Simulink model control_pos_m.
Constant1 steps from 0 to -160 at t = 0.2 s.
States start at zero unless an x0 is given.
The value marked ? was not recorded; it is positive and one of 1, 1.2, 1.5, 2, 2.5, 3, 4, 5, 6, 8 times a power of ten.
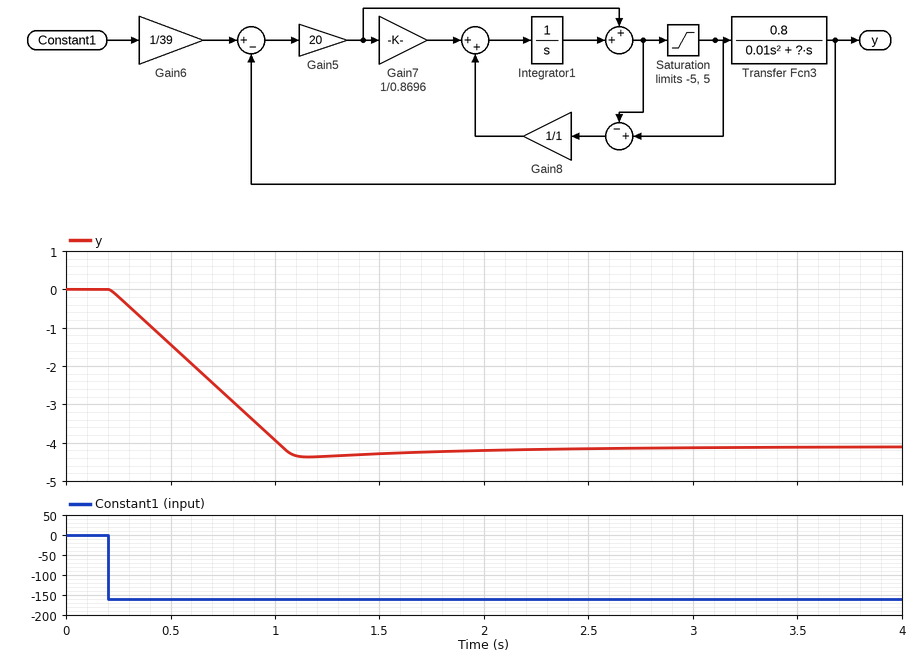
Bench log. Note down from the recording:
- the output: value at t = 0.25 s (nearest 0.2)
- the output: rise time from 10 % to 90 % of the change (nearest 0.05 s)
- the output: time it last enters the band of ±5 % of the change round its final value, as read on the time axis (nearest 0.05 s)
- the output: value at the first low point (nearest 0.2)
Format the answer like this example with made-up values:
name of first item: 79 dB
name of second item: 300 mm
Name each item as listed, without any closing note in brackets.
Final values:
the output: value at t = 0.25 s: -0.2
the output: rise time from 10 % to 90 % of the change: 0.65 s
the output: time it last enters the band of ±5 % of the change round its final value, as read on the time axis: 1.40 s
the output: value at the first low point: -4.4
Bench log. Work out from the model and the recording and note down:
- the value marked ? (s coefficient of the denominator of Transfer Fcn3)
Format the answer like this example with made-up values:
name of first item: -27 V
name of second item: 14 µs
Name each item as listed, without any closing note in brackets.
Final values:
the value marked ?: 0.8
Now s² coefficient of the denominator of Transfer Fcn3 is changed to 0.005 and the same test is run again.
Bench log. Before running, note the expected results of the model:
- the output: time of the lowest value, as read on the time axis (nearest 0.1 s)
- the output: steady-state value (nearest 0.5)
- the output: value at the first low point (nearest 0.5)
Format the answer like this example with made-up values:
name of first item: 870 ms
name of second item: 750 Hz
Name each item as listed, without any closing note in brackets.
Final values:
the output: time of the lowest value, as read on the time axis: 1.2 s
the output: steady-state value: -4.0
the output: value at the first low point: -4.5
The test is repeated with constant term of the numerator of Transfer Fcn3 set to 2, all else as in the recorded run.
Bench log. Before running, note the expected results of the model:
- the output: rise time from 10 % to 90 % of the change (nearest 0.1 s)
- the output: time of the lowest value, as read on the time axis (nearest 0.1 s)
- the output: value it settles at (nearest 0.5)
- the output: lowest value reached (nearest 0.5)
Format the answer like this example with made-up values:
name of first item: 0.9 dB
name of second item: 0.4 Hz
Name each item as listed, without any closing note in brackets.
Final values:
the output: rise time from 10 % to 90 % of the change: 0.3 s
the output: time of the lowest value, as read on the time axis: 0.6 s
the output: value it settles at: -4.0
the output: lowest value reached: -4.5
